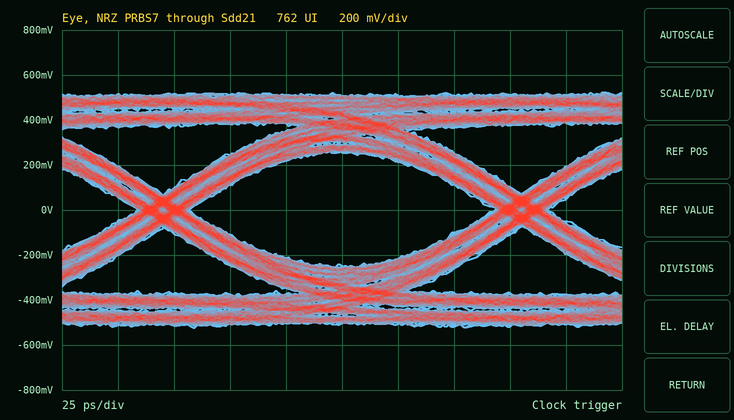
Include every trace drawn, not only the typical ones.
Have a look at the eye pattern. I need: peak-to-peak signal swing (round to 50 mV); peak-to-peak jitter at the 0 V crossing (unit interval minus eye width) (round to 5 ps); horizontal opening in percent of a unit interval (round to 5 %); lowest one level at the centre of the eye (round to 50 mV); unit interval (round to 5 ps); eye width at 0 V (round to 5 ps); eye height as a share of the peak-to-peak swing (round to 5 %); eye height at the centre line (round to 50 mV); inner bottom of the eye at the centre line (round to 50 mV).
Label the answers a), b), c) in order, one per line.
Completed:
a) 1.05 V
b) 25 ps
c) 85 %
d) 250 mV
e) 160 ps
f) 135 ps
g) 50 %
h) 500 mV
i) -250 mV
